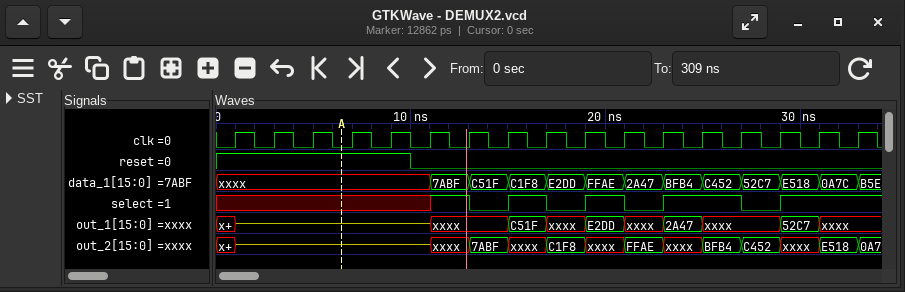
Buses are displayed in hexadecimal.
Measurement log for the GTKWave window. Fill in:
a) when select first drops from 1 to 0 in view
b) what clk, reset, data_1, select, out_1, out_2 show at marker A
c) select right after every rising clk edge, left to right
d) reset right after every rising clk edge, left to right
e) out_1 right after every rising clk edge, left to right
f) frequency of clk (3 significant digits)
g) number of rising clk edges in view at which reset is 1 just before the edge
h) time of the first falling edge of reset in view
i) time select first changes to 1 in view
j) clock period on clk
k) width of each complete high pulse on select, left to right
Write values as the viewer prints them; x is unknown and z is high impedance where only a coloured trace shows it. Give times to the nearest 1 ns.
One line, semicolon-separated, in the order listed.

13 ns; clk=0, reset=1, data_1=xxxx, select=x, out_1=z, out_2=z; x x x x x 1 0 1 0 1 0 1 1 0 1 1 1; 1 1 1 1 1 0 0 0 0 0 0 0 0 0 0 0 0; z, z, z, z, z, xxxx, xxxx, C51F, xxxx, E2DD, xxxx, 2A47, xxxx, xxxx, 52C7, xxxx, xxxx; 500 MHz; 5; 10 ns; 11 ns; 2 ns; 2 ns, 2 ns, 4 ns
